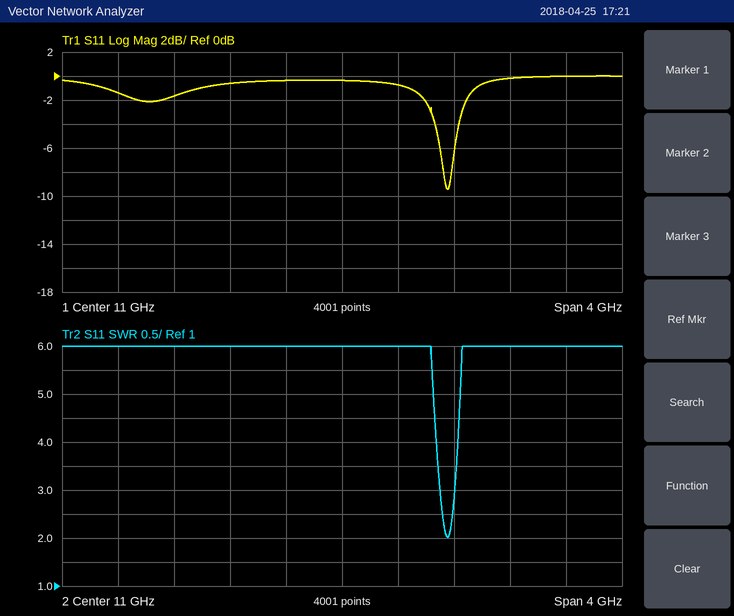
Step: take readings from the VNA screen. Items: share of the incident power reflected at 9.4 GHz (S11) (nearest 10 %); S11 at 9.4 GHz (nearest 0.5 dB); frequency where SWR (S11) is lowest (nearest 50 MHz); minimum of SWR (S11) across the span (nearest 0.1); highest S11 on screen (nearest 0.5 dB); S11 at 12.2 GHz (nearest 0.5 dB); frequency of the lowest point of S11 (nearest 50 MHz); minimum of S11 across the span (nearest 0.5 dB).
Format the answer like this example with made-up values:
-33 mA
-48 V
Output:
70 %
-1.5 dB
11.75 GHz
2.0
0.0 dB
0.0 dB
11.75 GHz
-9.5 dB
